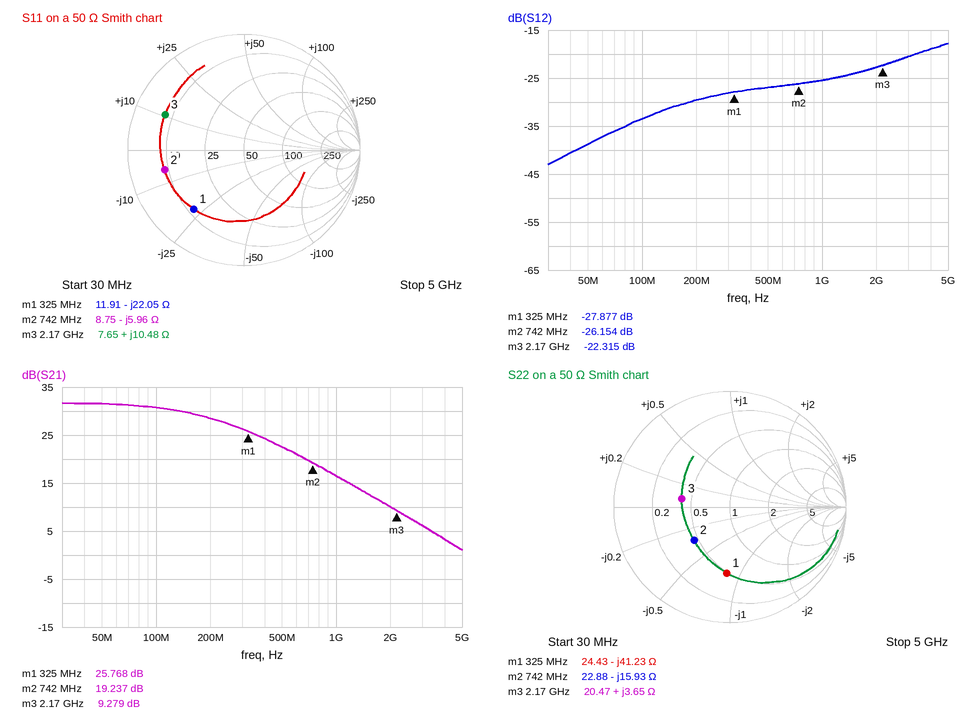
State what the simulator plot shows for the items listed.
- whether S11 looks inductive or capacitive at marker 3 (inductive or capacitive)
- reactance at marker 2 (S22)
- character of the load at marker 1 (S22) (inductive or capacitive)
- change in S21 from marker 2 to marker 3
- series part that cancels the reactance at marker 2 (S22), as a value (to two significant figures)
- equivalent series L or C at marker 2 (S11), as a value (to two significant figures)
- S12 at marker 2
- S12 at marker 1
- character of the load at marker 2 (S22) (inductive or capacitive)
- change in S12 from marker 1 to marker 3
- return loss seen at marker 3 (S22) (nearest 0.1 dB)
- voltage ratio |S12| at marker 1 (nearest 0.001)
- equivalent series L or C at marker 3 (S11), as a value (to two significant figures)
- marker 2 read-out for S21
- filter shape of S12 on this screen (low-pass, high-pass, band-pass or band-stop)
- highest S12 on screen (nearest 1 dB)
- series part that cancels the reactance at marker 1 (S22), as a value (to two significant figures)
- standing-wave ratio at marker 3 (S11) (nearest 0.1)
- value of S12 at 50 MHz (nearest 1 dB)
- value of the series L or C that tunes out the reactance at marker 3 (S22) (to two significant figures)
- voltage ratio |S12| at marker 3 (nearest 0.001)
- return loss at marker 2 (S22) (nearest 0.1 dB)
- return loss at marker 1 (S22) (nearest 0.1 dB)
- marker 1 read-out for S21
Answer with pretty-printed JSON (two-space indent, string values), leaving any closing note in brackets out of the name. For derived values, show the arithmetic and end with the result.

{
  "whether S11 looks inductive or capacitive at marker 3": "inductive",
  "reactance at marker 2": "-15.93 Ω",
  "character of the load at marker 1 (S22)": "capacitive",
  "change in S21 from marker 2 to marker 3": "9.279 − (19.237) = -9.958 dB",
  "series part that cancels the reactance at marker 2 (S22), as a value": "L = 15.93 Ω/(2π × 742 MHz) ≈ 3.4 nH",
  "equivalent series L or C at marker 2 (S11), as a value": "C = 1/(2π × 742 MHz × 5.96 Ω) ≈ 36 pF",
  "S12 at marker 2": "-26.154 dB",
  "S12 at marker 1": "-27.877 dB",
  "character of the load at marker 2 (S22)": "capacitive",
  "change in S12 from marker 1 to marker 3": "-22.315 − (-27.877) = 5.562 dB",
  "return loss seen at marker 3 (S22)": "7.5 dB",
  "voltage ratio |S12| at marker 1": "10^(-27.877/20) ≈ 0.040",
  "equivalent series L or C at marker 3 (S11), as a value": "L = 10.48 Ω/(2π × 2.17 GHz) ≈ 769 pH, so 770 pH to two significant figures",
  "marker 2 read-out for S21": "19.237 dB",
  "filter shape of S12 on this screen": "high-pass",
  "highest S12 on screen": "-18 dB",
  "series part that cancels the reactance at marker 1 (S22), as a value": "L = 41.23 Ω/(2π × 325 MHz) ≈ 20 nH",
  "standing-wave ratio at marker 3 (S11)": "6.8",
  "value of S12 at 50 MHz": "-39 dB",
  "value of the series L or C that tunes out the reactance at marker 3 (S22)": "C = 1/(2π × 2.17 GHz × 3.65 Ω) ≈ 20 pF",
  "voltage ratio |S12| at marker 3": "10^(-22.315/20) ≈ 0.077",
  "return loss at marker 2 (S22)": "7.5 dB",
  "return loss at marker 1 (S22)": "4.9 dB",
  "marker 1 read-out for S21": "25.768 dB"
}
